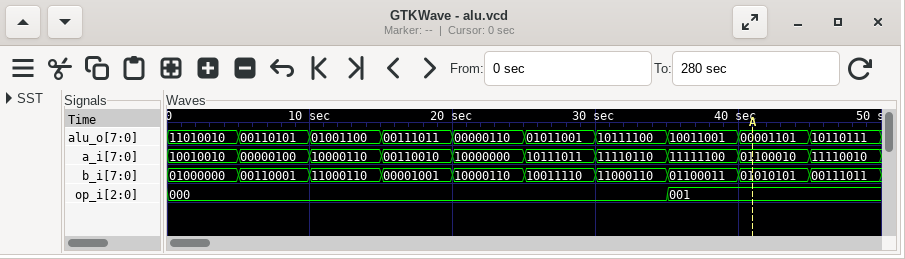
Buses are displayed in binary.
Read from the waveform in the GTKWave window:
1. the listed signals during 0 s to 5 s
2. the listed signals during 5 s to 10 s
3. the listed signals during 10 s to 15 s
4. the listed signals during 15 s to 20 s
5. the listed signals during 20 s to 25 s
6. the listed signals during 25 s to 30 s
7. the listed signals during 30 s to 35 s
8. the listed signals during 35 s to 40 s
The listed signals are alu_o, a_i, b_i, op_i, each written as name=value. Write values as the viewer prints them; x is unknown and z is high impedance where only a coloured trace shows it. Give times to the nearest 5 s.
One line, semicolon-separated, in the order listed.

alu_o=11010010, a_i=10010010, b_i=01000000, op_i=000; alu_o=00110101, a_i=00000100, b_i=00110001, op_i=000; alu_o=01001100, a_i=10000110, b_i=11000110, op_i=000; alu_o=00111011, a_i=00110010, b_i=00001001, op_i=000; alu_o=00000110, a_i=10000000, b_i=10000110, op_i=000; alu_o=01011001, a_i=10111011, b_i=10011110, op_i=000; alu_o=10111100, a_i=11110110, b_i=11000110, op_i=000; alu_o=10011001, a_i=11111100, b_i=01100011, op_i=001
